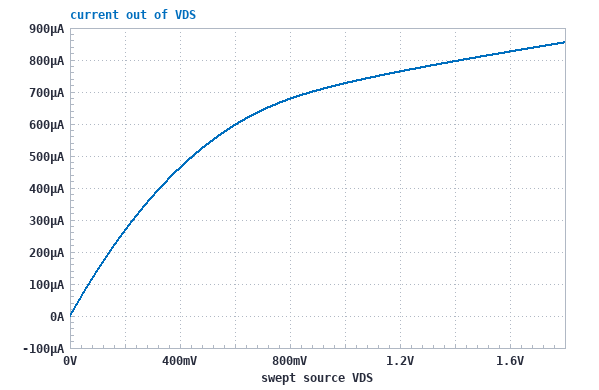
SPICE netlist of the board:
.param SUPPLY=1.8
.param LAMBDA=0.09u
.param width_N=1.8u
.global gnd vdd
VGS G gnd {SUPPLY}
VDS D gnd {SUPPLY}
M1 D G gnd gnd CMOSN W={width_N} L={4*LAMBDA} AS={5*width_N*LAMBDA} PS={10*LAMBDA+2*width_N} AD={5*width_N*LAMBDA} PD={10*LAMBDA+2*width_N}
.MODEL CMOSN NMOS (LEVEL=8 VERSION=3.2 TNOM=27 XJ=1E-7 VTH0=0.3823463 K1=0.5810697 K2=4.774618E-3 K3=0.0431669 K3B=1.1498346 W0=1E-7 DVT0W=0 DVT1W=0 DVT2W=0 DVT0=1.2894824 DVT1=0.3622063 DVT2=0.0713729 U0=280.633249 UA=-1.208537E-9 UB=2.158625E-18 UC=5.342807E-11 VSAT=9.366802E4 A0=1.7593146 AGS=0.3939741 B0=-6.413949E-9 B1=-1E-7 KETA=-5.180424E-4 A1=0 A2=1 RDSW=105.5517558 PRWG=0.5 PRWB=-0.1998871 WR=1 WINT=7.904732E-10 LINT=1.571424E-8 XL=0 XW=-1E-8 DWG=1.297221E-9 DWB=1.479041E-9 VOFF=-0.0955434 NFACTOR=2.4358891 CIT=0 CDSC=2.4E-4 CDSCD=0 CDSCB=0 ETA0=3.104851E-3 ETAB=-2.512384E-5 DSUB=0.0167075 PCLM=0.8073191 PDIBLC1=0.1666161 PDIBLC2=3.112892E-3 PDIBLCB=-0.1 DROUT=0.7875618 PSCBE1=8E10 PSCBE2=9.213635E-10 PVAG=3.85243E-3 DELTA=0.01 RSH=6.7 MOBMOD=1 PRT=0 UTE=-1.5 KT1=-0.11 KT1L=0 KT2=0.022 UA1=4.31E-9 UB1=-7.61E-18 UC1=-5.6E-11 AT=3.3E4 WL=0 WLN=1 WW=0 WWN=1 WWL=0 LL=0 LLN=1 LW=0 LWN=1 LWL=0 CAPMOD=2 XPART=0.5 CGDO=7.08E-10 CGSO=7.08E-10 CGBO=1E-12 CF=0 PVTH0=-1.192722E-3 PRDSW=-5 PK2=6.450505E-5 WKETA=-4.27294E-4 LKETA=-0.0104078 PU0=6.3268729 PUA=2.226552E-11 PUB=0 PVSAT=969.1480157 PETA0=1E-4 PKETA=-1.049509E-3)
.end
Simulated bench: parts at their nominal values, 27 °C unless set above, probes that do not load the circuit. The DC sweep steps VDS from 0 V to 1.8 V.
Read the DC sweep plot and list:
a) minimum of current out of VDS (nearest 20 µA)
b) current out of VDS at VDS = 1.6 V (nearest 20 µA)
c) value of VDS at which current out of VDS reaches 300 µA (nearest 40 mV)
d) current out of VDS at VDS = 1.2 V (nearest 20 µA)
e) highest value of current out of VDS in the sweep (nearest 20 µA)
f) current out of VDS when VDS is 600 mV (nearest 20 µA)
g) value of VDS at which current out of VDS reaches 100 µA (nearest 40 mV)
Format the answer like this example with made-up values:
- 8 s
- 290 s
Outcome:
- 0 A
- 820 µA
- 240 mV
- 760 µA
- 860 µA
- 600 µA
- 80 mV
